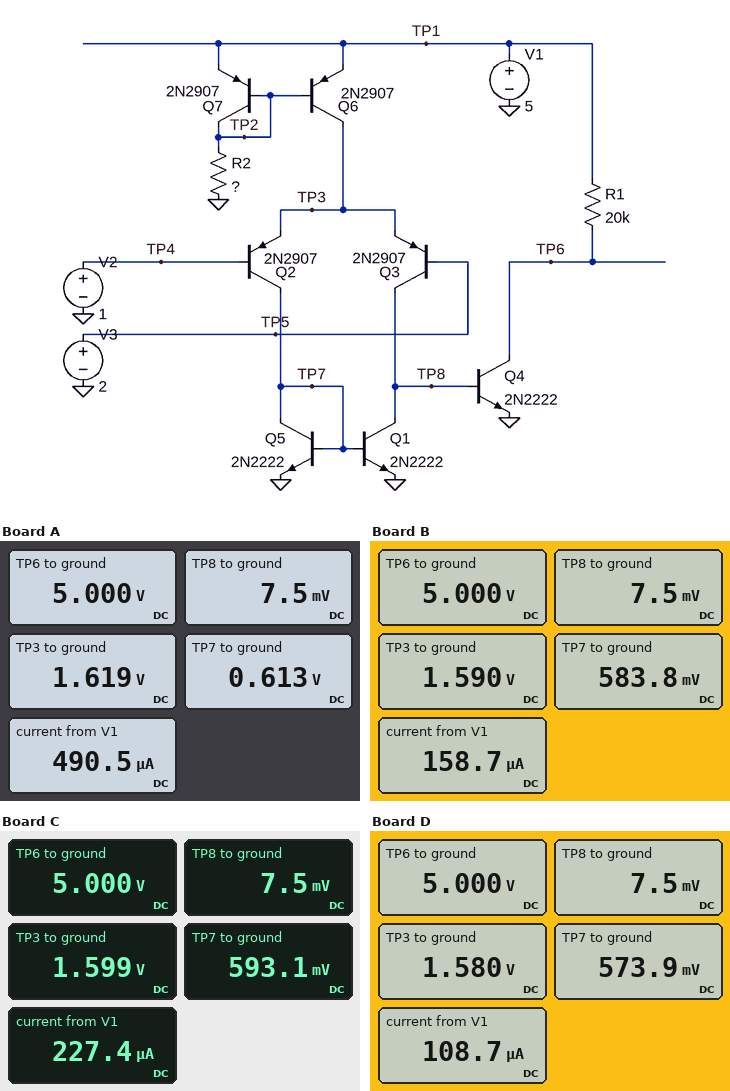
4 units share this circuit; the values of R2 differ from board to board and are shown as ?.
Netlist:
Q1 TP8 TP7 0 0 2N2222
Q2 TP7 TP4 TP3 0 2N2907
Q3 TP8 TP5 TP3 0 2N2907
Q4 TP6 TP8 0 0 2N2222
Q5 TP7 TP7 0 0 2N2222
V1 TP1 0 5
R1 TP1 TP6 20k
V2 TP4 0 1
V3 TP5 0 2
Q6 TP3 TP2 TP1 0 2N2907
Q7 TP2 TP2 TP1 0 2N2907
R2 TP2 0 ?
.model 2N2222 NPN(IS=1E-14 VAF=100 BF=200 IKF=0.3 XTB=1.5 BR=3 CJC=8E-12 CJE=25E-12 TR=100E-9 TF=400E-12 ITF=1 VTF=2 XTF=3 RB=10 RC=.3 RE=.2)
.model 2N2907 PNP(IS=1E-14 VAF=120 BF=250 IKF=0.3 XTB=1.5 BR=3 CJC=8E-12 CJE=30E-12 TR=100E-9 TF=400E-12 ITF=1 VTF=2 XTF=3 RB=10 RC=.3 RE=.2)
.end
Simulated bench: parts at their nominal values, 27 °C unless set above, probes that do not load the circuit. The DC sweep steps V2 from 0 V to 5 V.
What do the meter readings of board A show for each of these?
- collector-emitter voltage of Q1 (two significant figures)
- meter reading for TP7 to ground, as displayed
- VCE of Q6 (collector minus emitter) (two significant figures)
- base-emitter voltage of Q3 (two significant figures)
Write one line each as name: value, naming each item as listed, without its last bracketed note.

collector-emitter voltage of Q1: 7.5 mV
meter reading for TP7 to ground, as displayed: 0.613 V
VCE of Q6 (collector minus emitter): -3.4 V
base-emitter voltage of Q3: 380 mV
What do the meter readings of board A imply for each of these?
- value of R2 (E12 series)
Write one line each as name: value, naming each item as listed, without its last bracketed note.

value of R2: 18 kΩ
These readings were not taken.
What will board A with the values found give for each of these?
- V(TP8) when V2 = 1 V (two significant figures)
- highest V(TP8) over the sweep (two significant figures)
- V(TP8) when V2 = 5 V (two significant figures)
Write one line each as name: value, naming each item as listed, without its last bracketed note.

V(TP8) when V2 = 1 V: 7.5 mV
highest V(TP8) over the sweep: 660 mV
V(TP8) when V2 = 5 V: 660 mV
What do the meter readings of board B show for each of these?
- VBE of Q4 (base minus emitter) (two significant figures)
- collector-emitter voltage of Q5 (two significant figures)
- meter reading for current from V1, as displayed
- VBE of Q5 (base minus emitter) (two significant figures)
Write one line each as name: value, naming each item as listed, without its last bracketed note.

VBE of Q4 (base minus emitter): 7.5 mV
collector-emitter voltage of Q5: 580 mV
meter reading for current from V1, as displayed: 158.7 µA
VBE of Q5 (base minus emitter): 580 mV
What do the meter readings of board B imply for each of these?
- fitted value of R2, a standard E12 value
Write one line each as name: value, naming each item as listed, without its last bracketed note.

fitted value of R2, a standard E12 value: 56 kΩ
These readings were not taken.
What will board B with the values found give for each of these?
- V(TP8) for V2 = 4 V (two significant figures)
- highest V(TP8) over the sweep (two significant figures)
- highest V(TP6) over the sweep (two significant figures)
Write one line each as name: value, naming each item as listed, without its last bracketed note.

V(TP8) for V2 = 4 V: 640 mV
highest V(TP8) over the sweep: 640 mV
highest V(TP6) over the sweep: 5.0 V
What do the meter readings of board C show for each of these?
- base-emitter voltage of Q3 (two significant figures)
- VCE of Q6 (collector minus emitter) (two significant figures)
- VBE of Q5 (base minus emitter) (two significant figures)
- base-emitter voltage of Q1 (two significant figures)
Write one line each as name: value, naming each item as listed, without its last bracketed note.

base-emitter voltage of Q3: 400 mV
VCE of Q6 (collector minus emitter): -3.4 V
VBE of Q5 (base minus emitter): 590 mV
base-emitter voltage of Q1: 590 mV
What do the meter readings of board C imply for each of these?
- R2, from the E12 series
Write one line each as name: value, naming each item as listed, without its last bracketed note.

R2, from the E12 series: 39 kΩ
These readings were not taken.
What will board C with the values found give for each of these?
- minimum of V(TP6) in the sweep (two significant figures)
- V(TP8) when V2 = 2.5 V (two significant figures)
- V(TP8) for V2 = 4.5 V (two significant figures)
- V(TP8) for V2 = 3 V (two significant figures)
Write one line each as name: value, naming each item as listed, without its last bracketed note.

minimum of V(TP6) in the sweep: 19 mV
V(TP8) when V2 = 2.5 V: 650 mV
V(TP8) for V2 = 4.5 V: 650 mV
V(TP8) for V2 = 3 V: 650 mV
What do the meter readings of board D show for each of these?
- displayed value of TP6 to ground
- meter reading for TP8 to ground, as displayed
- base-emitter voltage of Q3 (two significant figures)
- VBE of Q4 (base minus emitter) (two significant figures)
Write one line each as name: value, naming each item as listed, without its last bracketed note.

displayed value of TP6 to ground: 5.000 V
meter reading for TP8 to ground, as displayed: 7.5 mV
base-emitter voltage of Q3: 420 mV
VBE of Q4 (base minus emitter): 7.5 mV
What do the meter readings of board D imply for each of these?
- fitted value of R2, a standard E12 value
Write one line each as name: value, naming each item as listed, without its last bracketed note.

fitted value of R2, a standard E12 value: 82 kΩ
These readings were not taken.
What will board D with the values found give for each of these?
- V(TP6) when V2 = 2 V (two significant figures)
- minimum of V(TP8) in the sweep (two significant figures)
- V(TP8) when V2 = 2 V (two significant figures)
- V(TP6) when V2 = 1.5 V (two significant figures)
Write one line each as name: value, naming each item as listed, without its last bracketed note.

V(TP6) when V2 = 2 V: 3.9 V
minimum of V(TP8) in the sweep: 7.5 mV
V(TP8) when V2 = 2 V: 580 mV
V(TP6) when V2 = 1.5 V: 5.0 V
